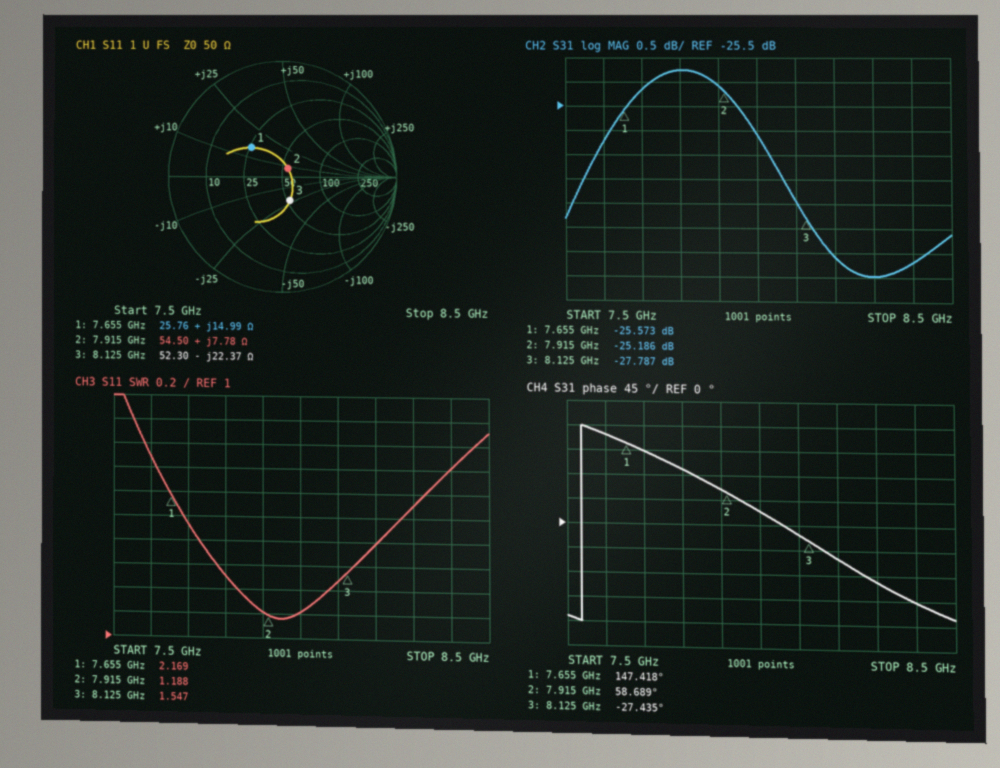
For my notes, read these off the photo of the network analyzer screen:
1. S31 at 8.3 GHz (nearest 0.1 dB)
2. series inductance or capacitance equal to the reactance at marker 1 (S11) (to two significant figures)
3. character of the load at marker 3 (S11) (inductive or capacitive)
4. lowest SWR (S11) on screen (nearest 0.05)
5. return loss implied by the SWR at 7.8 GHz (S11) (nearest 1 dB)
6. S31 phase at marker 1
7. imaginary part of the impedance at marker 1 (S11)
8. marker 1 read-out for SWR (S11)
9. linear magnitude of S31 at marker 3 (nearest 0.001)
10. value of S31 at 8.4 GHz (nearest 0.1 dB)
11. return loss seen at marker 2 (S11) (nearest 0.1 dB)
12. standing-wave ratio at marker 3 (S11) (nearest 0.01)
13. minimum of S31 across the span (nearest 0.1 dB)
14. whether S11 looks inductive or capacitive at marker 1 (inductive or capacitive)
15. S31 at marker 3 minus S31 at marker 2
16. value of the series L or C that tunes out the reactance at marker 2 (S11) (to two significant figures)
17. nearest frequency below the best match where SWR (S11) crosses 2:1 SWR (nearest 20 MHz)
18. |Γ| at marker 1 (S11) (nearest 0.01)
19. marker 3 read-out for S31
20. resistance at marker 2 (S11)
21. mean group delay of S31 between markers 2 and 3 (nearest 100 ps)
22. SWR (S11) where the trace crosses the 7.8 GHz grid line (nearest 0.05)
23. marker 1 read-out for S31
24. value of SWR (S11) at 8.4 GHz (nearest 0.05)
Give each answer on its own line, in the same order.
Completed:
-29.0 dB
310 pH
capacitive
1.15
14 dB
147.418°
+14.99 Ω
2.169
0.041
-28.7 dB
21.3 dB
1.55
-29.0 dB
inductive
-2.601 dB
2.6 pF
7.68 GHz
0.37
-27.787 dB
54.50 Ω
1.1 ns
1.50
-25.573 dB
2.40
